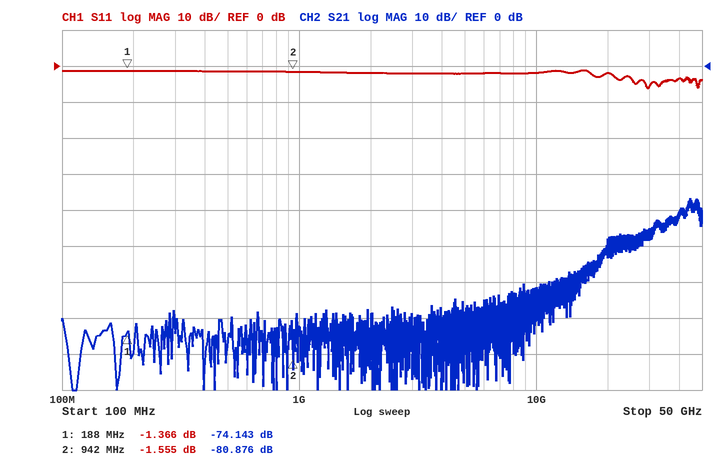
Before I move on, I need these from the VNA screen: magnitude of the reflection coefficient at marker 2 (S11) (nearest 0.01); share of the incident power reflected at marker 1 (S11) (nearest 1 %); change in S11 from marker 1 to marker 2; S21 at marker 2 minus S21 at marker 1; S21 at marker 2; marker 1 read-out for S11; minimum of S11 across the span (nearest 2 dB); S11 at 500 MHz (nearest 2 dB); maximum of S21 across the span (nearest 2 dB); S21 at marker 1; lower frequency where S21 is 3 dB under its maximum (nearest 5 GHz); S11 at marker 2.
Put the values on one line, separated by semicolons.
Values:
0.84; 73 %; -0.189 dB; -6.733 dB; -80.876 dB; -1.366 dB; -6 dB; -2 dB; -36 dB; -74.143 dB; 45 GHz; -1.555 dB
